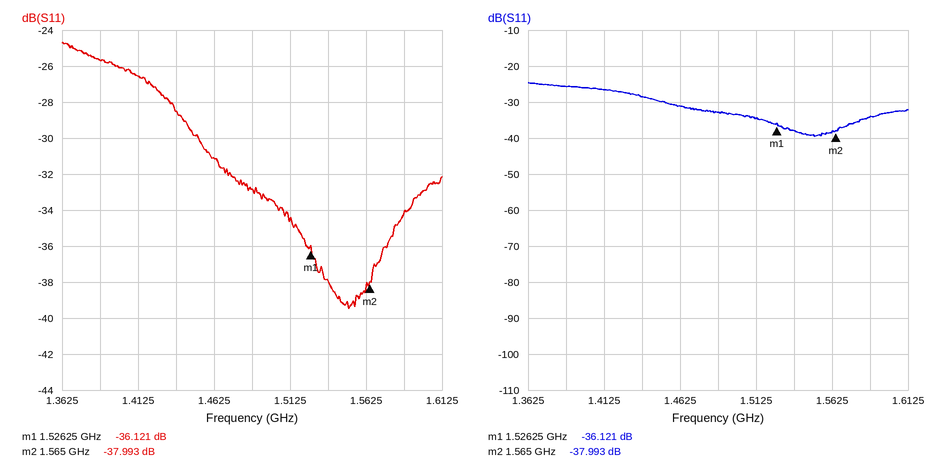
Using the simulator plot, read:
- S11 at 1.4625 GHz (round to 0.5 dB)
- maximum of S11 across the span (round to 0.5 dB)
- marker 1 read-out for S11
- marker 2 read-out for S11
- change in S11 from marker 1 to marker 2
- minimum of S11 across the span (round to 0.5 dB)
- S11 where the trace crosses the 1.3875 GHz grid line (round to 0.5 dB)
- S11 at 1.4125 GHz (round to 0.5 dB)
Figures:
-31.0 dB
-24.5 dB
-36.121 dB
-37.993 dB
-1.872 dB
-39.5 dB
-25.5 dB
-26.5 dB
